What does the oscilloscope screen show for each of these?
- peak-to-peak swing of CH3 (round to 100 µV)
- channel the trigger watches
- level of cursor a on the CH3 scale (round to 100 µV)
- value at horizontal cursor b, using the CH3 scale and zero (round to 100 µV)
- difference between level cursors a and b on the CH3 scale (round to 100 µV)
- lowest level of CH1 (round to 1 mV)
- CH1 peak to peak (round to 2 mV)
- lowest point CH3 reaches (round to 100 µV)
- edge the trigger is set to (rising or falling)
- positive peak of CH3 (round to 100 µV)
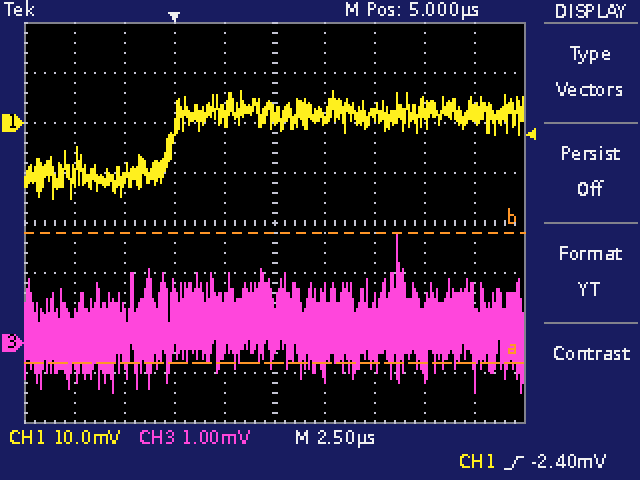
3.2 mV
CH1
-400 µV
2.2 mV
2.6 mV
-15 mV
22 mV
-1.0 mV
rising
2.2 mV
